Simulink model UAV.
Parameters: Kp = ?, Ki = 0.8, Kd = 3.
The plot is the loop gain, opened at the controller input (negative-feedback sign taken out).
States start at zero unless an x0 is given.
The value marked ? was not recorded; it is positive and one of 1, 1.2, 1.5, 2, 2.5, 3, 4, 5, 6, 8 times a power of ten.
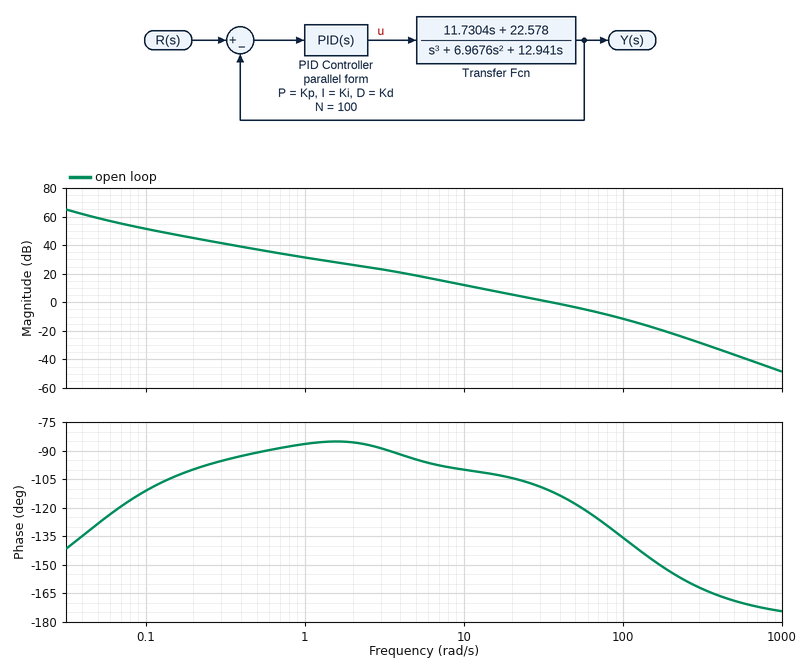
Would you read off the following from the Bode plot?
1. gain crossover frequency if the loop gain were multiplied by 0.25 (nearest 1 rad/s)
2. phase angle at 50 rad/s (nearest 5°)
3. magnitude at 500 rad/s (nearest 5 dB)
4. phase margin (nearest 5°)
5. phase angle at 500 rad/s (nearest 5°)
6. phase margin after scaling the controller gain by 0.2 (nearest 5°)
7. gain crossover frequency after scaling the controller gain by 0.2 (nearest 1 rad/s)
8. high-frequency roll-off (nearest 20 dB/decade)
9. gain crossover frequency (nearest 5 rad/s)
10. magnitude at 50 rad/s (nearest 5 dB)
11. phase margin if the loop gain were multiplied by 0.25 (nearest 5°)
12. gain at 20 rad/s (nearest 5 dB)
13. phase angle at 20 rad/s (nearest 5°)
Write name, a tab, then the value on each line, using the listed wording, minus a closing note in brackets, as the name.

gain crossover frequency if the loop gain were multiplied by 0.25	10 rad/s
phase angle at 50 rad/s	-120°
magnitude at 500 rad/s	-35 dB
phase margin	70°
phase angle at 500 rad/s	-170°
phase margin after scaling the controller gain by 0.2	80°
gain crossover frequency after scaling the controller gain by 0.2	8 rad/s
high-frequency roll-off	-40 dB/decade
gain crossover frequency	35 rad/s
magnitude at 50 rad/s	-5 dB
phase margin if the loop gain were multiplied by 0.25	80°
gain at 20 rad/s	5 dB
phase angle at 20 rad/s	-105°
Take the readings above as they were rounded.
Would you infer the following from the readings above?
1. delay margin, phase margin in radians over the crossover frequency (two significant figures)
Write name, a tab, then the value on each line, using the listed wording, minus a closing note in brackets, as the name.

delay margin, phase margin in radians over the crossover frequency	0.035 s
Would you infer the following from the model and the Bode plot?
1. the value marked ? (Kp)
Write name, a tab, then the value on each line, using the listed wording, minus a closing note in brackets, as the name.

the value marked ?	20
